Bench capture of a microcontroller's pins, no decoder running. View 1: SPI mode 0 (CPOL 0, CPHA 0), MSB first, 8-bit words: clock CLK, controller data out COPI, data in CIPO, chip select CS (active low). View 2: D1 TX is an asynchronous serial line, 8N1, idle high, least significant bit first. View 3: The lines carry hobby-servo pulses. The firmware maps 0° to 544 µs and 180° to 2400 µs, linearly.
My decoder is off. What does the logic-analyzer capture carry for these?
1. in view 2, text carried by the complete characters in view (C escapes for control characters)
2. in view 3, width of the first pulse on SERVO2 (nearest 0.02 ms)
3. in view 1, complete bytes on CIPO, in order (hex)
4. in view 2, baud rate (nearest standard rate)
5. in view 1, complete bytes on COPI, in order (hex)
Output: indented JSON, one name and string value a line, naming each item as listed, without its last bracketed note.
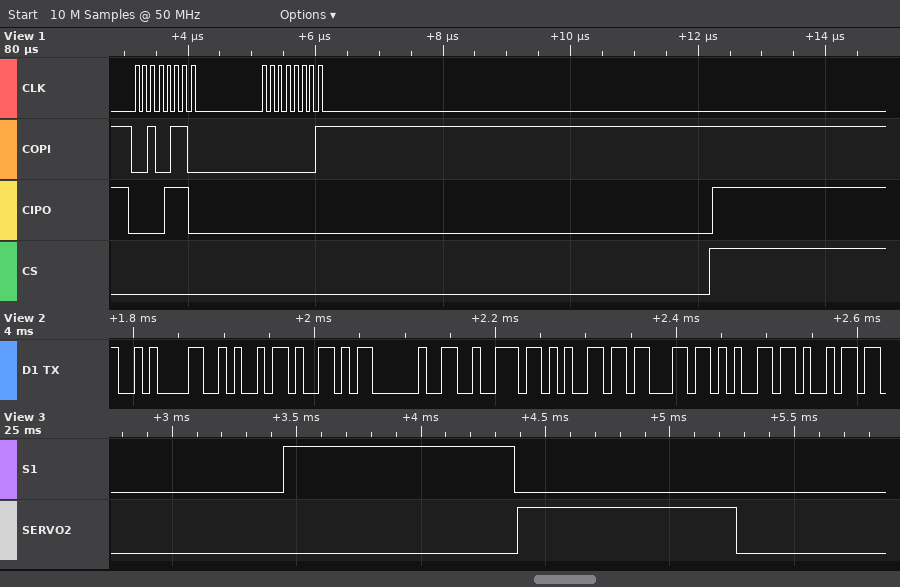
{
  "in view 2, text carried by the complete characters in view": "\"\\nJY recei\"",
  "in view 3, width of the first pulse on SERVO2": "0.88 ms",
  "in view 1, complete bytes on CIPO, in order": "0E 00",
  "in view 2, baud rate": "115200 baud",
  "in view 1, complete bytes on COPI, in order": "26 01"
}
